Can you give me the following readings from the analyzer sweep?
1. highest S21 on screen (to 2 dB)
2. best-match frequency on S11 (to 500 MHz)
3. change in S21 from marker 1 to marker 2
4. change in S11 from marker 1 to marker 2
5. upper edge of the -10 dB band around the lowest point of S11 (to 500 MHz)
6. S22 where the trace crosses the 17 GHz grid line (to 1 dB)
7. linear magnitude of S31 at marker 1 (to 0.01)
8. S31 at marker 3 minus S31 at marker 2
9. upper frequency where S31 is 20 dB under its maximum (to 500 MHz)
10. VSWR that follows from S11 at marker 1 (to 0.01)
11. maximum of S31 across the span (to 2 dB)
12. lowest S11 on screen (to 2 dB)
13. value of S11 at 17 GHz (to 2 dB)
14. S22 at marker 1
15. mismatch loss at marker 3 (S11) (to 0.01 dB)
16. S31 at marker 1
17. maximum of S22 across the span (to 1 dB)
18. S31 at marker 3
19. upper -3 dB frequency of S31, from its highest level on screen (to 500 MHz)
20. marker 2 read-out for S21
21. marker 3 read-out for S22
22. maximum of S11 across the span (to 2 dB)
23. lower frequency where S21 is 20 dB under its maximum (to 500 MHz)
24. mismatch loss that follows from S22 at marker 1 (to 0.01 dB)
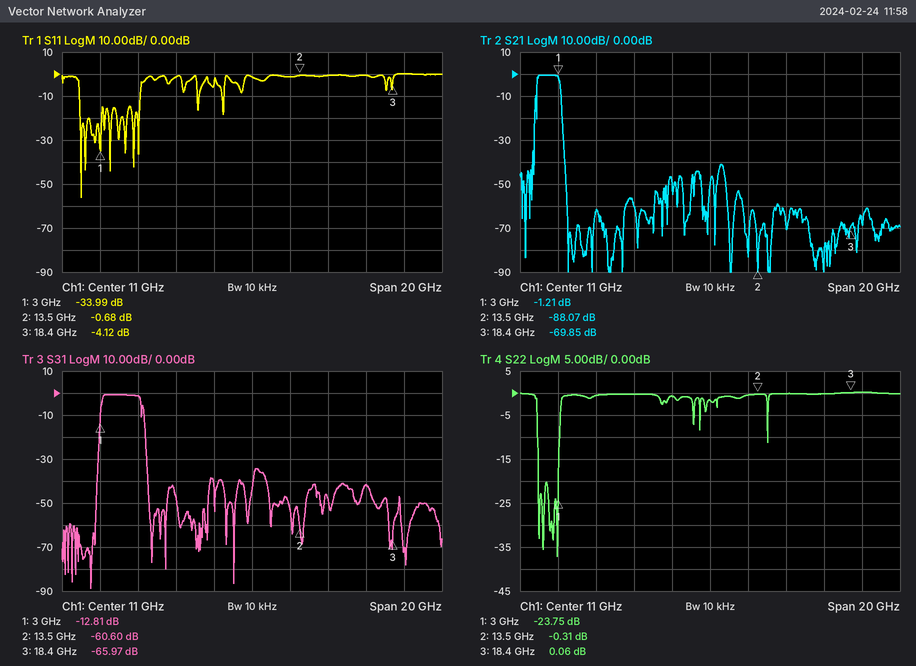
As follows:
0 dB
2.0 GHz
-86.86 dB
33.31 dB
5.0 GHz
0 dB
0.23
-5.37 dB
5.5 GHz
1.04
0 dB
-56 dB
0 dB
-23.75 dB
2.13 dB
-12.81 dB
0 dB
-65.97 dB
5.0 GHz
-88.07 dB
0.06 dB
0 dB
2.0 GHz
0.02 dB
